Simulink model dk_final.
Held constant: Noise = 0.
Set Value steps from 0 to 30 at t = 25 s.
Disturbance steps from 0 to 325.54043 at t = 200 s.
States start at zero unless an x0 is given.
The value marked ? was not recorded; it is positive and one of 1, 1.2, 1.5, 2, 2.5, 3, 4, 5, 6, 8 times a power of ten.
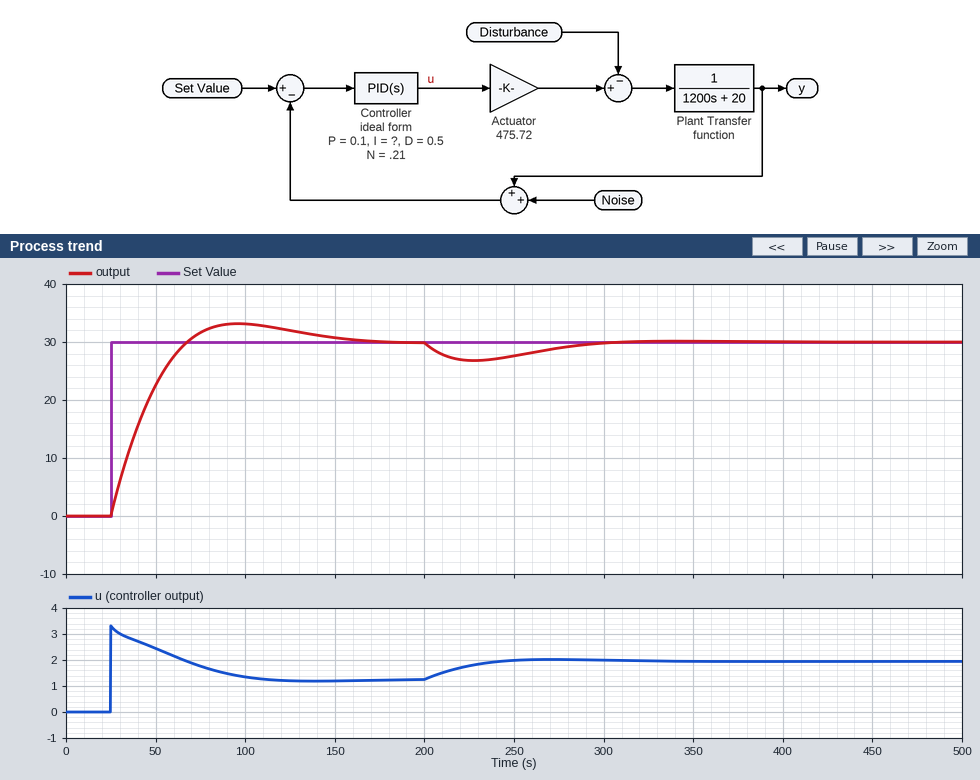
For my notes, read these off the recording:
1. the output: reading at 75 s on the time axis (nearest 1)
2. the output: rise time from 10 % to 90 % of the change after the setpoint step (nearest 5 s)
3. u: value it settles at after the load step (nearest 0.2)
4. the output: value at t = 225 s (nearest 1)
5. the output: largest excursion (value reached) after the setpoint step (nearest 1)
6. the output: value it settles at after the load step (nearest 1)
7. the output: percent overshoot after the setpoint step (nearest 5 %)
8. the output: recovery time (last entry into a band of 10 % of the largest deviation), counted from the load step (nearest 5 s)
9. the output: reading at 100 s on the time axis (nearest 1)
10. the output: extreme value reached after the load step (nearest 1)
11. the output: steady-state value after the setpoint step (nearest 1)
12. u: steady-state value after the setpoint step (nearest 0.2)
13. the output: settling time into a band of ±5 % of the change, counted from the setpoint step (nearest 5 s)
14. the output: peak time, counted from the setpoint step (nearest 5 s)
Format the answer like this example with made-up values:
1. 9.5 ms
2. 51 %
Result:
1. 32
2. 30 s
3. 2.0
4. 27
5. 33
6. 30
7. 10 %
8. 95 s
9. 33
10. 27
11. 30
12. 1.2
13. 110 s
14. 70 s
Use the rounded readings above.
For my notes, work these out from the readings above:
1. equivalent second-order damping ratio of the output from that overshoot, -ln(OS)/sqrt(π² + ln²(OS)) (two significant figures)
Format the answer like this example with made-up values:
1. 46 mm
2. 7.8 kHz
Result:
1. 0.59
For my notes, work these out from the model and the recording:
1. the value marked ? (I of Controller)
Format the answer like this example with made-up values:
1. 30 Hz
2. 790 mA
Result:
1. 0.04
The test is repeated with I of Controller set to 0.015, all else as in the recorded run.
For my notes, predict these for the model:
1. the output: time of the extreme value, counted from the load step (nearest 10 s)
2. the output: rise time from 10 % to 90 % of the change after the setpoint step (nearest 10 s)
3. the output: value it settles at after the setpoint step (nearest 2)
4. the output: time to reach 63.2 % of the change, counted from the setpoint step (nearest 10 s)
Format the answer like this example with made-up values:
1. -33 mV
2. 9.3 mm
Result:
1. 40 s
2. 60 s
3. 30
4. 30 s
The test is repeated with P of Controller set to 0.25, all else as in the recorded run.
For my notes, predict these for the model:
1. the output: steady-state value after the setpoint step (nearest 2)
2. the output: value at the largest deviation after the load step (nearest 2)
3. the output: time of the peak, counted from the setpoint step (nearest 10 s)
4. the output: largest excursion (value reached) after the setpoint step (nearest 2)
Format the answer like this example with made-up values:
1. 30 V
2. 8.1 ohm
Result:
1. 30
2. 28
3. 40 s
4. 32
